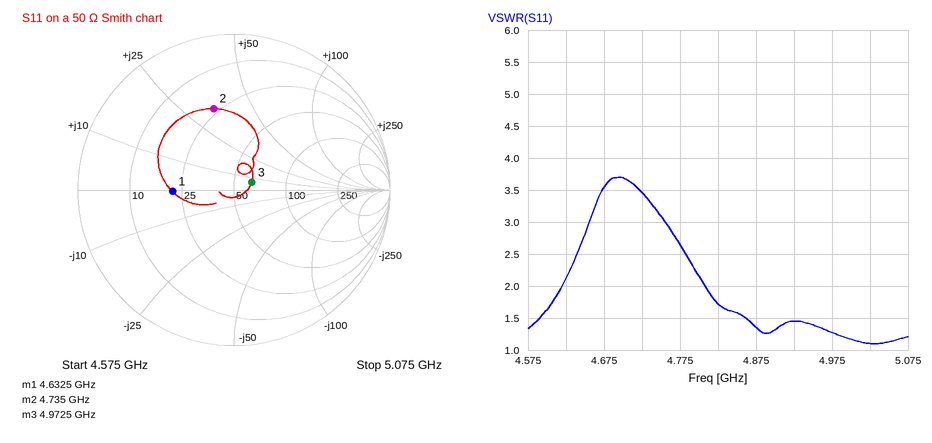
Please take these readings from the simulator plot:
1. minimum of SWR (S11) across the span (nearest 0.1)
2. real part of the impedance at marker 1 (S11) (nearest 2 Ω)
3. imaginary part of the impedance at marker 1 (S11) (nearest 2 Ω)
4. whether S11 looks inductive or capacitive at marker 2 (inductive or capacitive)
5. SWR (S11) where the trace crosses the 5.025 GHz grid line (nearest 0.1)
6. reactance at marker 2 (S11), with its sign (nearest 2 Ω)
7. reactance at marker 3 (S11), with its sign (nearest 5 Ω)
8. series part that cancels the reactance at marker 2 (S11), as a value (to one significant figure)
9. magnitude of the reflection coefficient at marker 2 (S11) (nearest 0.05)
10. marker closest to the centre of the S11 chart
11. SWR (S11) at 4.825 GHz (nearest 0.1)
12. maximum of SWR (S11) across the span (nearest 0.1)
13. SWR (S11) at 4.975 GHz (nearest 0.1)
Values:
1.1
22 Ω
0 Ω
inductive
1.1
+34 Ω
+5 Ω
1.0 pF
0.55
marker 3
1.7
3.7
1.3
